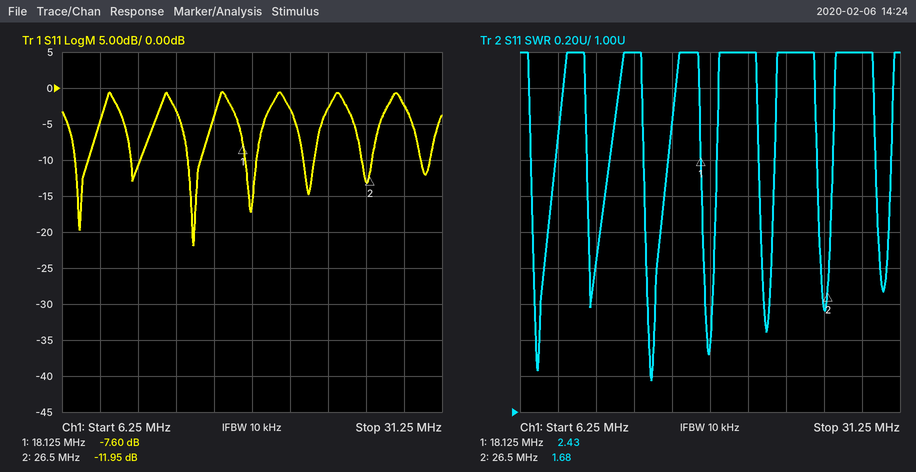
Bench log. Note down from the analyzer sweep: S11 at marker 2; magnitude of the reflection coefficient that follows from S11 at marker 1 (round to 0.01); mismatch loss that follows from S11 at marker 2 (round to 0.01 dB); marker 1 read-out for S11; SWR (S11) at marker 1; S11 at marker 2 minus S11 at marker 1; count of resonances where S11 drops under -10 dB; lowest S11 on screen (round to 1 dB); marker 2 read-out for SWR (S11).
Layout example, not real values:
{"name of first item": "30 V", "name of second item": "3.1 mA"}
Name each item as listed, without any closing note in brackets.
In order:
{"S11 at marker 2": "-11.95 dB", "magnitude of the reflection coefficient that follows from S11 at marker 1": "0.42", "mismatch loss that follows from S11 at marker 2": "0.29 dB", "marker 1 read-out for S11": "-7.60 dB", "SWR (S11) at marker 1": "2.43", "S11 at marker 2 minus S11 at marker 1": "-4.35 dB", "count of resonances where S11 drops under -10 dB": "7", "lowest S11 on screen": "-22 dB", "marker 2 read-out for SWR": "1.68"}
